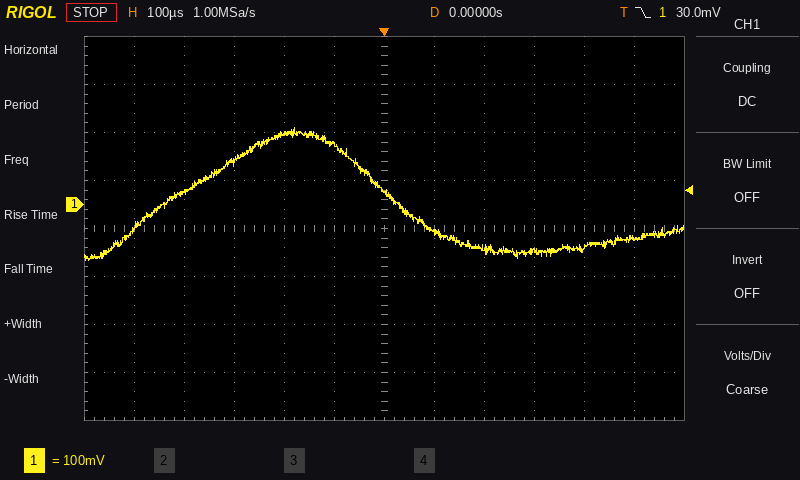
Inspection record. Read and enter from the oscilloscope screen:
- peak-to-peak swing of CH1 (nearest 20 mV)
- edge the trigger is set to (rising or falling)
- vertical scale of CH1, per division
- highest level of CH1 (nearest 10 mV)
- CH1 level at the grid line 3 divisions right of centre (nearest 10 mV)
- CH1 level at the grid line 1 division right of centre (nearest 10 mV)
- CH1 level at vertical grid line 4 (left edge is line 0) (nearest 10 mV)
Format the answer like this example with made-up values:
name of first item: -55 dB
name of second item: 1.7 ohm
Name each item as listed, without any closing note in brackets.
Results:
peak-to-peak swing of CH1: 280 mV
edge the trigger is set to: falling
vertical scale of CH1, per division: 100 mV
highest level of CH1: 160 mV
CH1 level at the grid line 3 divisions right of centre: -100 mV
CH1 level at the grid line 1 division right of centre: -60 mV
CH1 level at vertical grid line 4 (left edge is line 0): 150 mV
